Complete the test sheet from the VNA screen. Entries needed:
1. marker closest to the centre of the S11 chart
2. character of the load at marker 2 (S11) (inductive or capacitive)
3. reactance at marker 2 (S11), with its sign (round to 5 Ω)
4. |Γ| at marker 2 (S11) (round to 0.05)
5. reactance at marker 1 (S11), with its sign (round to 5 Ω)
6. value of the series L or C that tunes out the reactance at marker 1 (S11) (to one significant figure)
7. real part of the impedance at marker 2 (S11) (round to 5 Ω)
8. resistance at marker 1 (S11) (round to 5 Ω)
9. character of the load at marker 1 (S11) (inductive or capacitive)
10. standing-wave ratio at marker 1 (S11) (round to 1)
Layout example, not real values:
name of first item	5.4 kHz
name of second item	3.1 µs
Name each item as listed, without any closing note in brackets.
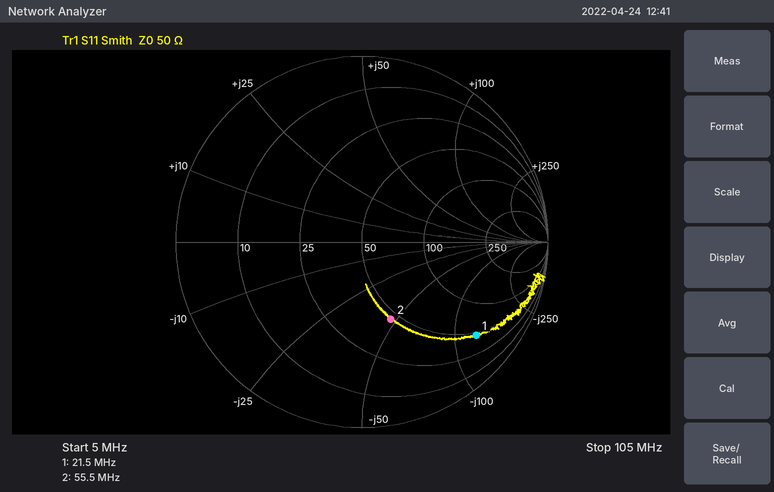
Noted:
marker closest to the centre of the S11 chart	marker 2
character of the load at marker 2 (S11)	capacitive
reactance at marker 2 (S11), with its sign	-45 Ω
|Γ| at marker 2 (S11)	0.45
reactance at marker 1 (S11), with its sign	-125 Ω
value of the series L or C that tunes out the reactance at marker 1 (S11)	900 nH
real part of the impedance at marker 2 (S11)	45 Ω
resistance at marker 1 (S11)	45 Ω
character of the load at marker 1 (S11)	capacitive
standing-wave ratio at marker 1 (S11)	9
